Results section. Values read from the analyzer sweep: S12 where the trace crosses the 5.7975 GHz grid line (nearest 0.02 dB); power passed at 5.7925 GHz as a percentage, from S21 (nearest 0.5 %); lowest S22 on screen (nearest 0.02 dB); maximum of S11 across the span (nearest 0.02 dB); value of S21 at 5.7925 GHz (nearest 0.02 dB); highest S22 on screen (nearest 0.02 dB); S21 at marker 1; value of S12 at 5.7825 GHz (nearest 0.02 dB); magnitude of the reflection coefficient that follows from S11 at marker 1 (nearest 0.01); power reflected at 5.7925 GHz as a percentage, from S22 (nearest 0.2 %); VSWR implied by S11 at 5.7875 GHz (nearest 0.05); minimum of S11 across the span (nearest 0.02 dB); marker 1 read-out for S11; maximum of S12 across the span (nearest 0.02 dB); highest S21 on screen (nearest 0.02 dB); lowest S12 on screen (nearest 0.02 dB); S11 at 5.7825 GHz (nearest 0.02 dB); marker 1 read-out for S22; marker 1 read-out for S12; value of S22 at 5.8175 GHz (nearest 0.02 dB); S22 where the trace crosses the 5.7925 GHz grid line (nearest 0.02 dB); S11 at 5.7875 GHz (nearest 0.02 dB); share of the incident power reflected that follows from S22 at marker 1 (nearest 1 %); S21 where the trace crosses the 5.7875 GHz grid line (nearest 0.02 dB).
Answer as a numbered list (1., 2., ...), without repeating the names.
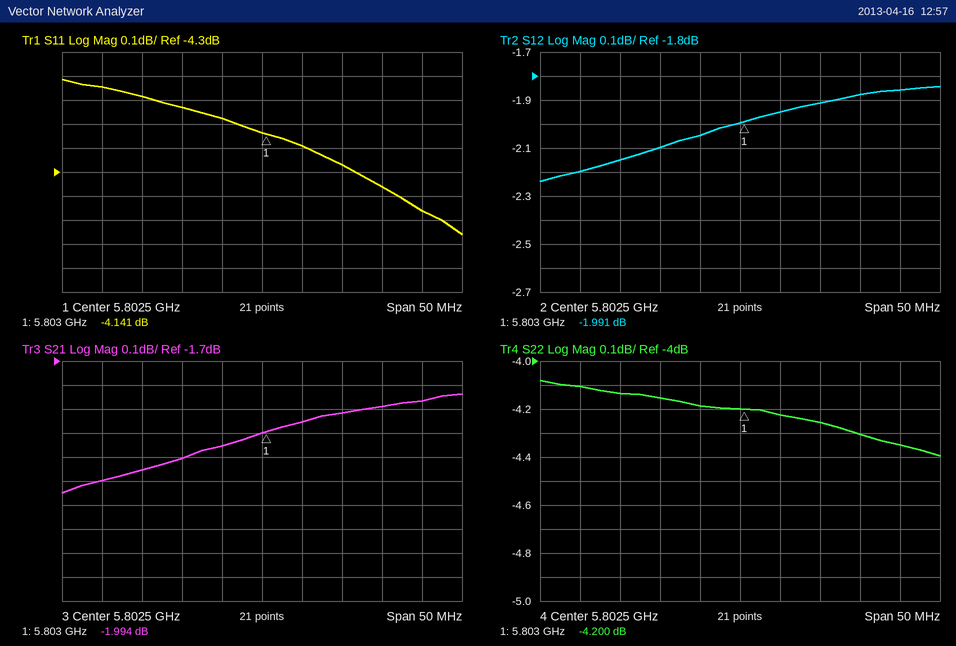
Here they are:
1. -2.04 dB
2. 61.5 %
3. -4.40 dB
4. -3.92 dB
5. -2.10 dB
6. -4.08 dB
7. -1.994 dB
8. -2.20 dB
9. 0.62
10. 38.4 %
11. 4.45
12. -4.56 dB
13. -4.141 dB
14. -1.84 dB
15. -1.84 dB
16. -2.24 dB
17. -3.94 dB
18. -4.200 dB
19. -1.991 dB
20. -4.30 dB
21. -4.16 dB
22. -3.98 dB
23. 38 %
24. -2.16 dB
